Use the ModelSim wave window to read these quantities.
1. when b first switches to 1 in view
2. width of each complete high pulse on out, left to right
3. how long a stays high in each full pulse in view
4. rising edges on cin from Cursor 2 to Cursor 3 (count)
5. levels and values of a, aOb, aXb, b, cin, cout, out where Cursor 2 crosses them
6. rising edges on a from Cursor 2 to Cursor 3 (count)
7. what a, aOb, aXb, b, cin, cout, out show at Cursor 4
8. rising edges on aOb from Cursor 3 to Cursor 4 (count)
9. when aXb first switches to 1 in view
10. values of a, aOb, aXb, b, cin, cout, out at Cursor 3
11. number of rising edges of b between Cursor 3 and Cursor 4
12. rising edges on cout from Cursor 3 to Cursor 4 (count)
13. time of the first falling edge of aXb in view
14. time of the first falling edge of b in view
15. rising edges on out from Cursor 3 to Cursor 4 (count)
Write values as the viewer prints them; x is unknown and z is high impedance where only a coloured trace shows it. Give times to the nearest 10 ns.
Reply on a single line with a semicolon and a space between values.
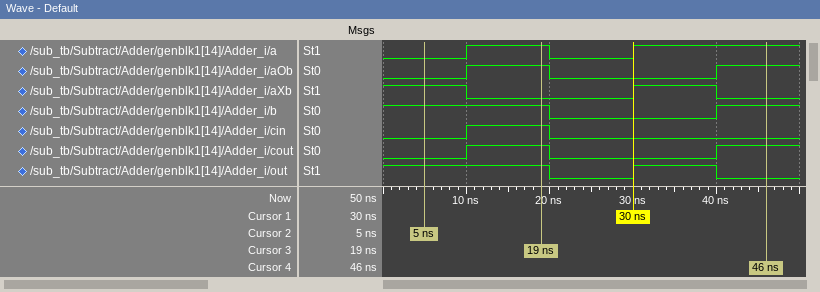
40 ns; 10 ns; 10 ns; 1; a=0, aOb=0, aXb=1, b=1, cin=0, cout=0, out=1; 1; a=1, aOb=1, aXb=0, b=1, cin=0, cout=1, out=0; 1; 30 ns; a=1, aOb=1, aXb=0, b=1, cin=1, cout=1, out=1; 1; 1; 10 ns; 20 ns; 1
